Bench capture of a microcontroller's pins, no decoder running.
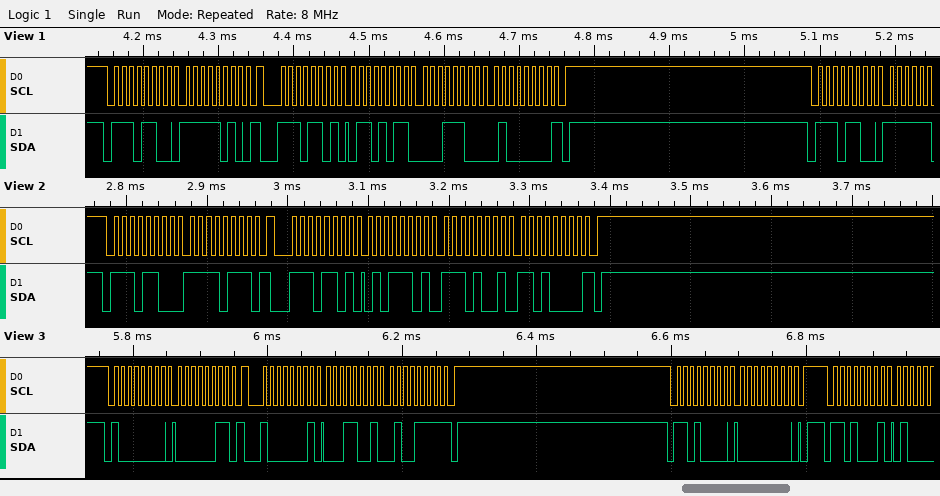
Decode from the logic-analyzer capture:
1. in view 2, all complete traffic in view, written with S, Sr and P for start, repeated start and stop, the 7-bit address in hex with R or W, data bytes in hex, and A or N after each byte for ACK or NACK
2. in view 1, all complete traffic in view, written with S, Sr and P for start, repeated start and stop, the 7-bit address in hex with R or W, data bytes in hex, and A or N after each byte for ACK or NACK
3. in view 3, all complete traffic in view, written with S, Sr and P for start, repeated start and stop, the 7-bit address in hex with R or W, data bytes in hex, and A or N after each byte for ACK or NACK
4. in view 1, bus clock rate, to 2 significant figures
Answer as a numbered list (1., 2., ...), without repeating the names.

1. S 76W A F7 A Sr 76R A 5D A E9 A D0 N P
2. S 76W A FA A Sr 76R A 6B A 1C A 40 N P S 76W A
3. S 40W A 03 A Sr 40R A 19 A 4F N P S 68W A 00 A P S 68R A
4. 100 kHz
